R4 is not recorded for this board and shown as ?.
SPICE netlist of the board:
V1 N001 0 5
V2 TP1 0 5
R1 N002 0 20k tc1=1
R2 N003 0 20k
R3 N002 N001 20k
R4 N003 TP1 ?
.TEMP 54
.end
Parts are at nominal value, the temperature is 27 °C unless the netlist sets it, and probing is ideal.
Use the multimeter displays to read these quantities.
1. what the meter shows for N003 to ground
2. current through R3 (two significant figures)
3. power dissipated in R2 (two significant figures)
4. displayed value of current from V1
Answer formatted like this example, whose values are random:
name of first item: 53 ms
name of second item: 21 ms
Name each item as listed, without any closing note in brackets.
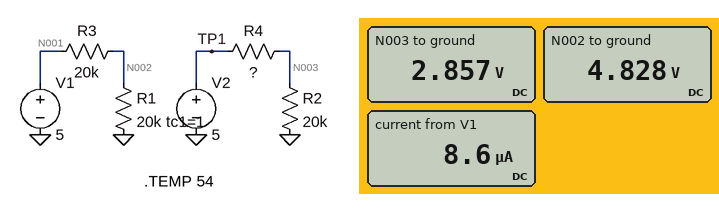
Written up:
what the meter shows for N003 to ground: 2.857 V
current through R3: 8.6 µA
power dissipated in R2: 410 µW
displayed value of current from V1: 8.6 µA
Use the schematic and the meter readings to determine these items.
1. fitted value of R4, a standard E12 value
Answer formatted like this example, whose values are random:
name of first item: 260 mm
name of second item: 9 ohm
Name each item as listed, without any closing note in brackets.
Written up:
fitted value of R4, a standard E12 value: 15 kΩ
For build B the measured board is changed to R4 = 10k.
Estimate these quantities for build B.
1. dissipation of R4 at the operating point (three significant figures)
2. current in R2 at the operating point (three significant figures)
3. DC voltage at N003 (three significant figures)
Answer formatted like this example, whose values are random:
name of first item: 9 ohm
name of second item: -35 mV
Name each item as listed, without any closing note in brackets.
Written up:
dissipation of R4 at the operating point: 278 µW
current in R2 at the operating point: 167 µA
DC voltage at N003: 3.33 V
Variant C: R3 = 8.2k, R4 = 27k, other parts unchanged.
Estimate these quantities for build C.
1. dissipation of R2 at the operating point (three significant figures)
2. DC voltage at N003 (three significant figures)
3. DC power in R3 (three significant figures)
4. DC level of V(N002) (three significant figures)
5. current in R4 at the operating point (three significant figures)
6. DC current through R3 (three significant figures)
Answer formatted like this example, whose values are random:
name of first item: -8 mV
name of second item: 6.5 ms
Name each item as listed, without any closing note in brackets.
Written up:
dissipation of R2 at the operating point: 226 µW
DC voltage at N003: 2.13 V
DC power in R3: 635 nW
DC level of V(N002): 4.93 V
current in R4 at the operating point: 106 µA
DC current through R3: 8.80 µA
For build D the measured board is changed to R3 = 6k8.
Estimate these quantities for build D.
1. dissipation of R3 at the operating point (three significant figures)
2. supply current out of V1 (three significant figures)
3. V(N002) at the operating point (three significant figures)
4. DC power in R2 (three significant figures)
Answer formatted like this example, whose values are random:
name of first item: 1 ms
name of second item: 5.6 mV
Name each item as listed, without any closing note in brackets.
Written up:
dissipation of R3 at the operating point: 529 nW
supply current out of V1: 8.82 µA
V(N002) at the operating point: 4.94 V
DC power in R2: 408 µW
